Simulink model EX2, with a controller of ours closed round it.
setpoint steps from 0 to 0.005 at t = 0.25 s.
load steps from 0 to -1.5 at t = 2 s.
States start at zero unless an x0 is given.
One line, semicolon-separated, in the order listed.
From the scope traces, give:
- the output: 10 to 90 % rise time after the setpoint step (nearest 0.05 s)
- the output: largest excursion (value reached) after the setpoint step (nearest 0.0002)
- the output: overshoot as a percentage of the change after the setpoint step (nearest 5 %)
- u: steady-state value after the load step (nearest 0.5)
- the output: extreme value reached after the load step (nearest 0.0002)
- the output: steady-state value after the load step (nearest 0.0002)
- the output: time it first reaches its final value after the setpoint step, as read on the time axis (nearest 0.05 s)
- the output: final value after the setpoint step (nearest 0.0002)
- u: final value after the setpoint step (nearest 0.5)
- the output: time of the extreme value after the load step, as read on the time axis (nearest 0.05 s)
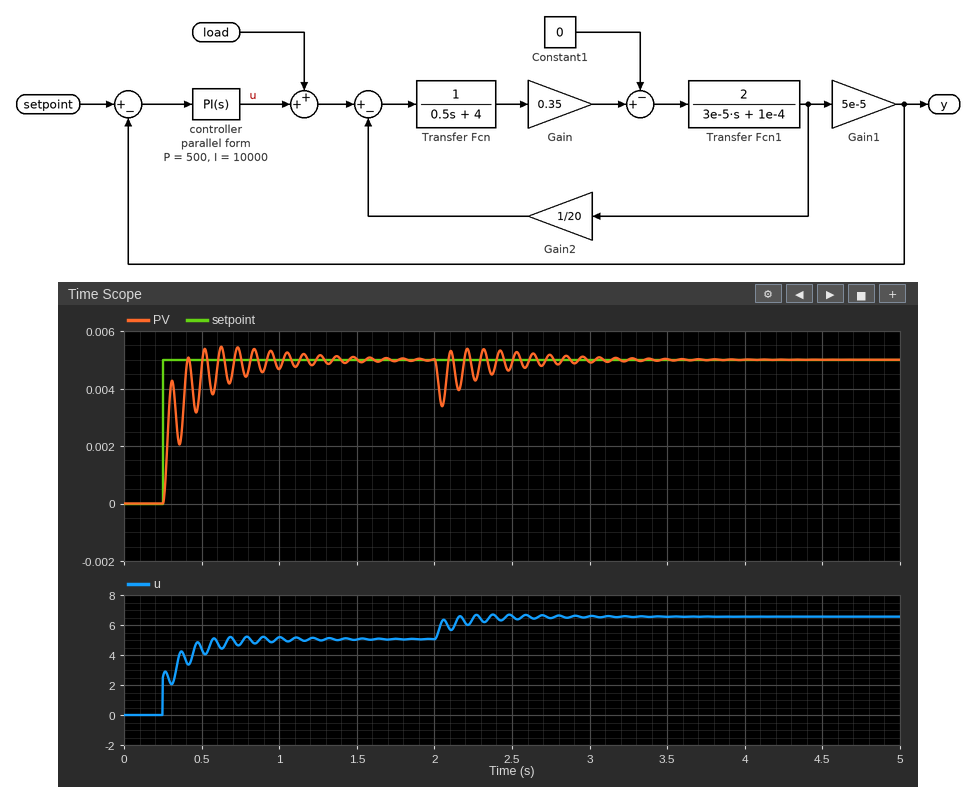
0.15 s; 0.0054; 10 %; 6.5; 0.0034; 0.0050; 0.40 s; 0.0050; 5.0; 2.05 s
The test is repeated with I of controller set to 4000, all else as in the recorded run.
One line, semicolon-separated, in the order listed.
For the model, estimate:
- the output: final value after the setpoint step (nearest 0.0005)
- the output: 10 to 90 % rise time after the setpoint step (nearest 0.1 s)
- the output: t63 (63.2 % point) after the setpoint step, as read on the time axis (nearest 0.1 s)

0.0050; 0.7 s; 0.3 s
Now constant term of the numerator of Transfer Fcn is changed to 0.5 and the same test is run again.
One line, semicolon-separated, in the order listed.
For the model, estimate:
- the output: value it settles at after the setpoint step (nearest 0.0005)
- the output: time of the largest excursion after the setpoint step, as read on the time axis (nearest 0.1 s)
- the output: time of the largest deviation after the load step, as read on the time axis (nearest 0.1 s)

0.0050; 0.6 s; 2.1 s
